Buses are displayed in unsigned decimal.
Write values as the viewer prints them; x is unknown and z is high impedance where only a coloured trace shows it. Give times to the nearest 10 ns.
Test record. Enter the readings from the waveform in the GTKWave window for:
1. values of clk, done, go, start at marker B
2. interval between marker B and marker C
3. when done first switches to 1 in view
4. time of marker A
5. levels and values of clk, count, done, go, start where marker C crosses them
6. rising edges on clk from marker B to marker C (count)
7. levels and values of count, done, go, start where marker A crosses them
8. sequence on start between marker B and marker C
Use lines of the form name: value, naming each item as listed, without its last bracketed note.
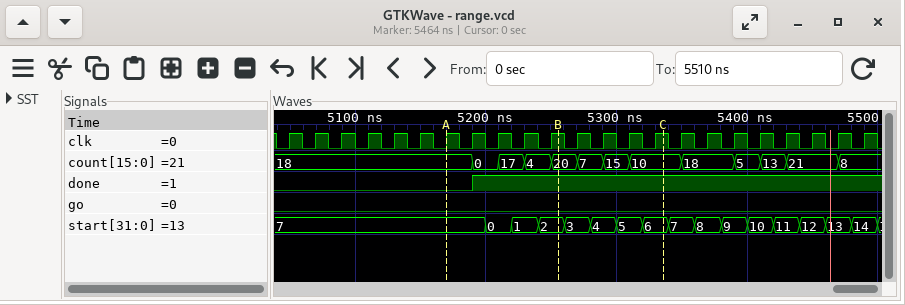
values of clk, done, go, start at marker B: clk=1, done=1, go=0, start=2
interval between marker B and marker C: 80 ns
when done first switches to 1 in view: 5190 ns
time of marker A: 5170 ns
levels and values of clk, count, done, go, start where marker C crosses them: clk=1, count=10, done=1, go=0, start=6
rising edges on clk from marker B to marker C: 4
levels and values of count, done, go, start where marker A crosses them: count=18, done=0, go=0, start=7
sequence on start between marker B and marker C: 2, 3, 4, 5, 6
